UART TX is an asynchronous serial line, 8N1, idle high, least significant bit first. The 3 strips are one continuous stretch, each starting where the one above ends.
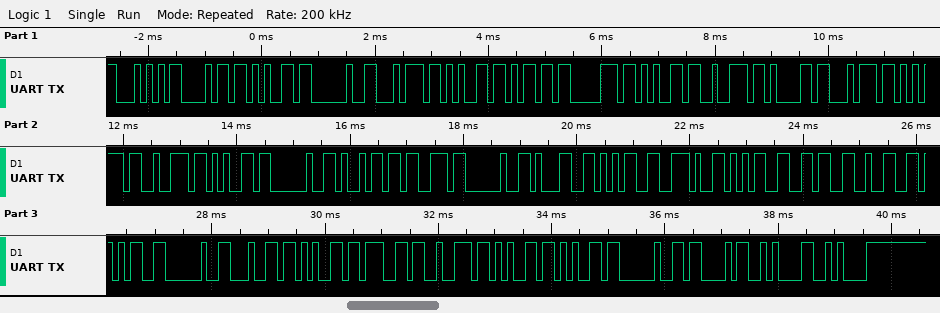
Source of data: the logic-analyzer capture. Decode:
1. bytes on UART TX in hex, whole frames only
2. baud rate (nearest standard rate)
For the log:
54 68 65 20 74 65 6D 70 65 72 61 74 75 72 65 20 69 73 20 31 35 2E 35 36 32 35 20 64 65 67 72 65 65 20 43 0A 0A
9600 baud
